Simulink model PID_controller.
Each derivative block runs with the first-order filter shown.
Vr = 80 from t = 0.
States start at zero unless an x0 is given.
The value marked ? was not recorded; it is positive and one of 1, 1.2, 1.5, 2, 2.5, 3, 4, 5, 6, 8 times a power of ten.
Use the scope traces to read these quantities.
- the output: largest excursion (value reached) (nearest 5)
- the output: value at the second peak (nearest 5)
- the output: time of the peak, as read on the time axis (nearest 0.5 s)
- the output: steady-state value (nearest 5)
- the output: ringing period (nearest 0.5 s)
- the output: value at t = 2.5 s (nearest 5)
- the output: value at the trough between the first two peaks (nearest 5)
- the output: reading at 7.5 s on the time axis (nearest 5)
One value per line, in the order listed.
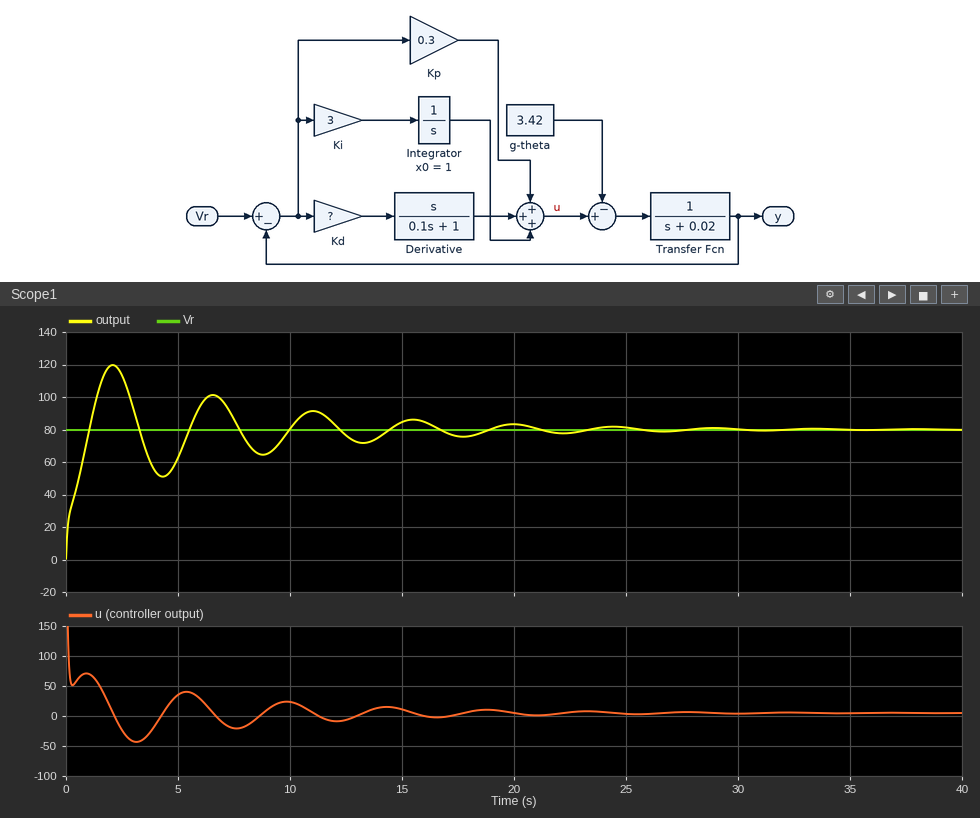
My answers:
120
100
2.0 s
80
4.5 s
115
50
85
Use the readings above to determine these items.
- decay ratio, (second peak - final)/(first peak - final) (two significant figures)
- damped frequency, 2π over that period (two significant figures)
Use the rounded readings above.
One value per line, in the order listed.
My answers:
0.50
1.4 rad/s
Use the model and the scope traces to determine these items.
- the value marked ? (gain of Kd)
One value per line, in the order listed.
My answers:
0.5
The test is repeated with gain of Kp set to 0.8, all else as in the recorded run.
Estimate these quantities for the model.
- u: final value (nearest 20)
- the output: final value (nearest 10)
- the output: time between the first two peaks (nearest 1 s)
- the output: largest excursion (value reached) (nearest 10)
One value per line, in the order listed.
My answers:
0
80
5 s
110
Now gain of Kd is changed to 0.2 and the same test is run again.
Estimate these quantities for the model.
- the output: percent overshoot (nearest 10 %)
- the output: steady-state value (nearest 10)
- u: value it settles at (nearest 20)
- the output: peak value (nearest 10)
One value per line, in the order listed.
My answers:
60 %
80
0
130
